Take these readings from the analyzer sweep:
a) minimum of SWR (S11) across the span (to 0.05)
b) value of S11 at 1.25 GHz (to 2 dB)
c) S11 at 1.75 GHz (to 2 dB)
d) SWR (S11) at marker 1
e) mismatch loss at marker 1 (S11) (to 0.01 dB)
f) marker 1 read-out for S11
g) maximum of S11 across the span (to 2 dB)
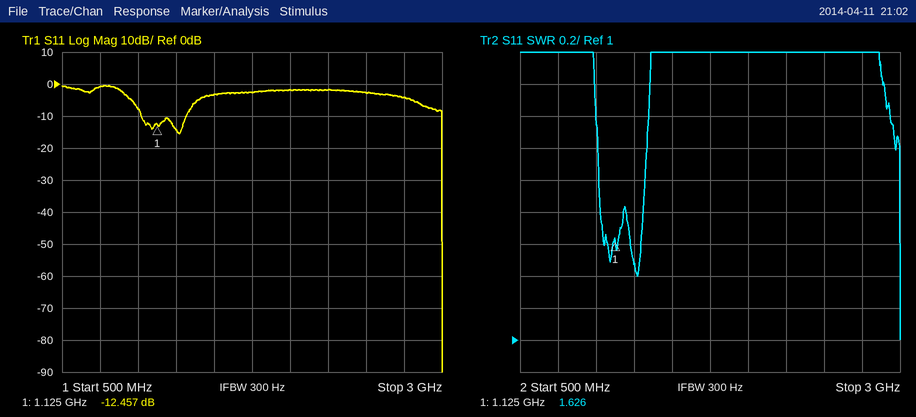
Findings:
1.00
-14 dB
-2 dB
1.626
0.25 dB
-12.457 dB
0 dB
